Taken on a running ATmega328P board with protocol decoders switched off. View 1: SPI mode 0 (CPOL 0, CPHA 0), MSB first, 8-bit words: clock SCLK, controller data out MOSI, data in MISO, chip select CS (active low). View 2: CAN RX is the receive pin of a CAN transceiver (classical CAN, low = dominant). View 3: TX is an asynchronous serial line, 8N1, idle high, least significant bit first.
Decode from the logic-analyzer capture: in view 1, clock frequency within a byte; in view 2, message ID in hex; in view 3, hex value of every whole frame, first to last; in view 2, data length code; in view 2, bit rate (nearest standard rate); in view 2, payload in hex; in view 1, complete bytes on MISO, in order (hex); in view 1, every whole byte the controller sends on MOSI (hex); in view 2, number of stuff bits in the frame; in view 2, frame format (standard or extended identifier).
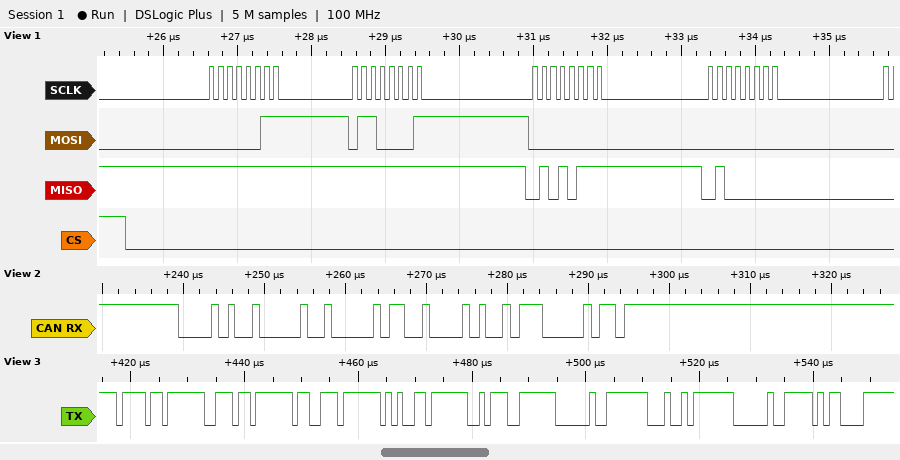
8 MHz
0x0A4
0x6F 0x6E 0x73 0x65 0x3A 0x20 0xA4 0x20 0x0D
2
1000 kbit/s
06 42
FF FF 57 40
03 61 00 00
3
standard
